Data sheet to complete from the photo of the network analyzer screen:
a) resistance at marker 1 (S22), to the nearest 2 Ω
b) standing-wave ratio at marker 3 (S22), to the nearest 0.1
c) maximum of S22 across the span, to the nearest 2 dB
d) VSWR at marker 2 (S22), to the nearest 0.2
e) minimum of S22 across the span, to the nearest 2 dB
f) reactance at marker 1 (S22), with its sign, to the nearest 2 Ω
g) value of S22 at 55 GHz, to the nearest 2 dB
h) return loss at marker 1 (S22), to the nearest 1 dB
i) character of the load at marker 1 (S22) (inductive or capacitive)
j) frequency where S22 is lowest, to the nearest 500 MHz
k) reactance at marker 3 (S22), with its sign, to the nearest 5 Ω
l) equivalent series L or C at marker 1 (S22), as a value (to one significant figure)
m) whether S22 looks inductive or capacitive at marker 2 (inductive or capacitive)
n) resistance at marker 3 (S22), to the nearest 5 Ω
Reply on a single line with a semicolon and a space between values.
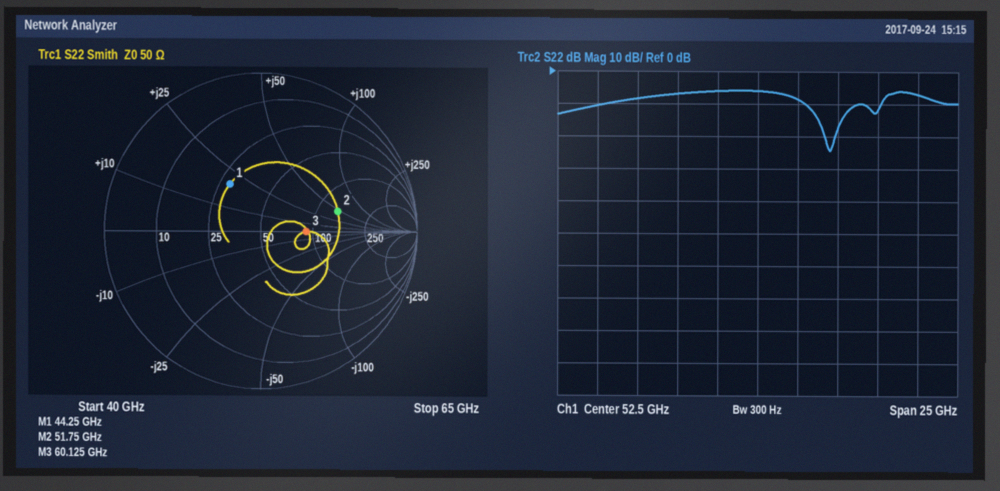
28 Ω; 1.8; -6 dB; 3.0; -24 dB; +20 Ω; -8 dB; 9 dB; inductive; 57.0 GHz; 0 Ω; 70 pH; inductive; 90 Ω
